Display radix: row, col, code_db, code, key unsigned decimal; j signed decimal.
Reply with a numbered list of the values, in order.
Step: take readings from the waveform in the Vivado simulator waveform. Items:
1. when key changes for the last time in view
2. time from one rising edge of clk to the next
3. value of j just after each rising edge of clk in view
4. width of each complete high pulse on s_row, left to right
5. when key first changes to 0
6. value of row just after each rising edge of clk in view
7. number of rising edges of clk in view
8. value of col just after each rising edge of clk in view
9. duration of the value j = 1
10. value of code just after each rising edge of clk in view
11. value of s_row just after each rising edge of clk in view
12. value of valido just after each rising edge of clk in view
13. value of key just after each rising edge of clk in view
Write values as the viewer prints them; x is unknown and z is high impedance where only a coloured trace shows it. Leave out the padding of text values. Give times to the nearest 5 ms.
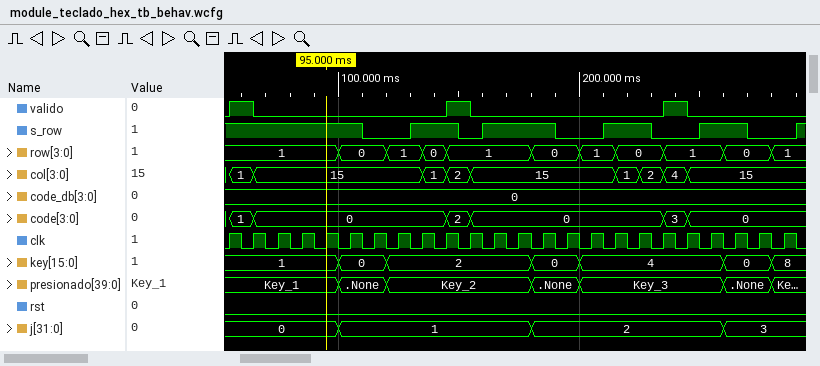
1. 280 ms
2. 10 ms
3. 0, 0, 0, 0, 0, 1, 1, 1, 1, 1, 1, 1, 1, 2, 2, 2, 2, 2, 2, 2, 2, 3, 3, 3
4. 20 ms, 30 ms, 20 ms, 20 ms
5. 100 ms
6. 1, 1, 1, 1, 1, 0, 0, 1, 0, 1, 1, 1, 1, 0, 0, 1, 0, 0, 1, 1, 1, 0, 0, 1
7. 24
8. 1, 15, 15, 15, 15, 15, 15, 15, 1, 2, 15, 15, 15, 15, 15, 15, 1, 2, 4, 15, 15, 15, 15, 15
9. 80 ms
10. 1, 0, 0, 0, 0, 0, 0, 0, 0, 2, 0, 0, 0, 0, 0, 0, 0, 0, 3, 0, 0, 0, 0, 0
11. 1 1 1 1 1 1 0 0 1 1 0 1 1 1 0 0 1 1 0 0 1 1 0 0
12. 1 0 0 0 0 0 0 0 0 1 0 0 0 0 0 0 0 0 1 0 0 0 0 0
13. 1, 1, 1, 1, 1, 0, 0, 2, 2, 2, 2, 2, 2, 0, 0, 4, 4, 4, 4, 4, 4, 0, 0, 8
